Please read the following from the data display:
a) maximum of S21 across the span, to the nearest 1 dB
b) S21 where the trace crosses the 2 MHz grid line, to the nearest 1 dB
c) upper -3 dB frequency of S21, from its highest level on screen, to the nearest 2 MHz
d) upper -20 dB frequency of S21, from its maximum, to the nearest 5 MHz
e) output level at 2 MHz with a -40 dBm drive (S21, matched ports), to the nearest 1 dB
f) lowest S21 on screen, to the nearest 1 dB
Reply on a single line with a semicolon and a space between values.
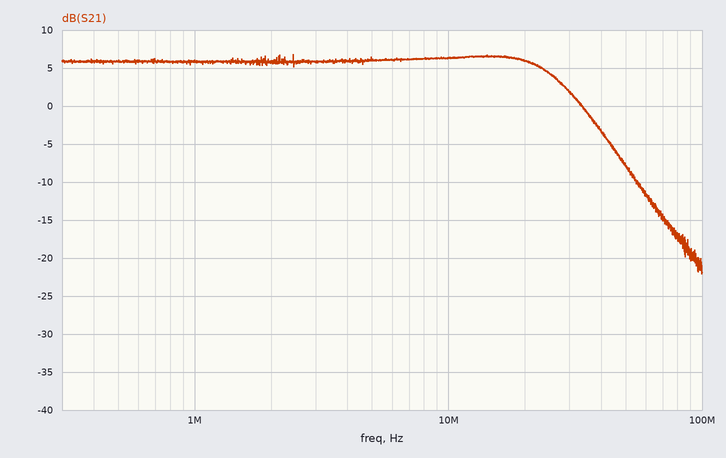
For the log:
7 dB; 6 dB; 26 MHz; 65 MHz; -34 dBm; -22 dB
